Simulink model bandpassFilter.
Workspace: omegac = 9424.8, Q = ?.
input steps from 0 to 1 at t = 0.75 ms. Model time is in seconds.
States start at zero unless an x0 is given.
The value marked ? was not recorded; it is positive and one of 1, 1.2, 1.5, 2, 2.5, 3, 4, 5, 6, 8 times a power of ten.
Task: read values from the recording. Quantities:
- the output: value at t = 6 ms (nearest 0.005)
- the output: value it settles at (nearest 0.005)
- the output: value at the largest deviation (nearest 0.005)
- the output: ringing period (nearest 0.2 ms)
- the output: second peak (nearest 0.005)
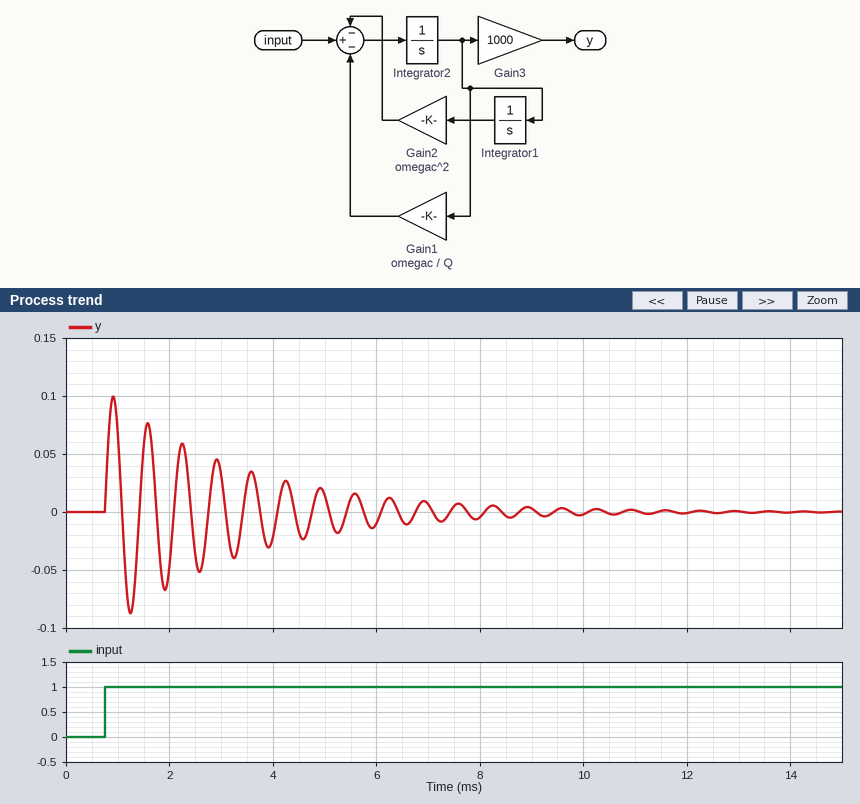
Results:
-0.010
0.000
0.100
0.6 ms
0.075
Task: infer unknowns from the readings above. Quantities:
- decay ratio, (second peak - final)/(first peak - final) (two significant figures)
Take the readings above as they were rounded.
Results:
0.75
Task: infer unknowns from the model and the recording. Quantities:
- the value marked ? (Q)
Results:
12
